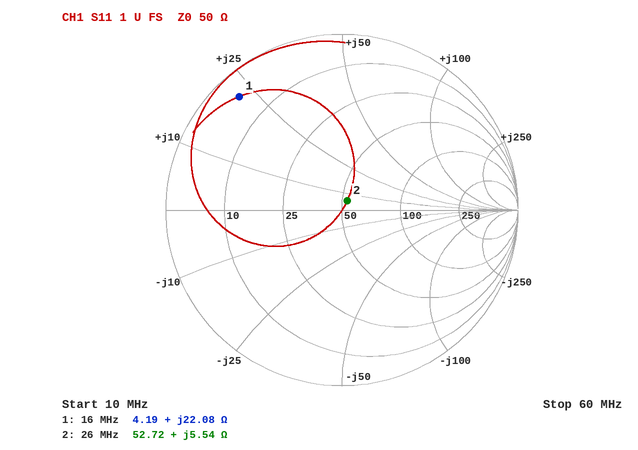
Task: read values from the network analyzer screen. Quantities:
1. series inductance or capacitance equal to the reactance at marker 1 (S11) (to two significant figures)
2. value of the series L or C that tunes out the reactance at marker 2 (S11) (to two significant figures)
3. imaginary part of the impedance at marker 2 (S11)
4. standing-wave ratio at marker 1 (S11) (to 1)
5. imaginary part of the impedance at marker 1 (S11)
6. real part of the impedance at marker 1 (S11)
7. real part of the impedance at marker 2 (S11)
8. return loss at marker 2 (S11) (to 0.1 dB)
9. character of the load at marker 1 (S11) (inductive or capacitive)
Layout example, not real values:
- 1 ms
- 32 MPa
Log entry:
- 220 nH
- 1.1 nF
- +5.54 Ω
- 14
- +22.08 Ω
- 4.19 Ω
- 52.72 Ω
- 24.4 dB
- inductive
